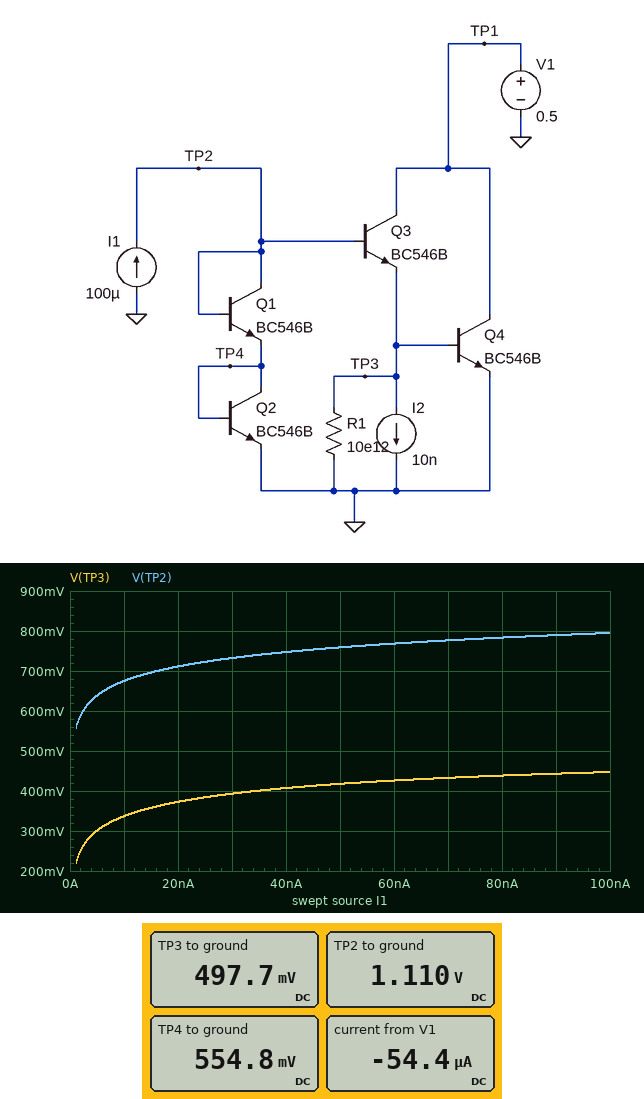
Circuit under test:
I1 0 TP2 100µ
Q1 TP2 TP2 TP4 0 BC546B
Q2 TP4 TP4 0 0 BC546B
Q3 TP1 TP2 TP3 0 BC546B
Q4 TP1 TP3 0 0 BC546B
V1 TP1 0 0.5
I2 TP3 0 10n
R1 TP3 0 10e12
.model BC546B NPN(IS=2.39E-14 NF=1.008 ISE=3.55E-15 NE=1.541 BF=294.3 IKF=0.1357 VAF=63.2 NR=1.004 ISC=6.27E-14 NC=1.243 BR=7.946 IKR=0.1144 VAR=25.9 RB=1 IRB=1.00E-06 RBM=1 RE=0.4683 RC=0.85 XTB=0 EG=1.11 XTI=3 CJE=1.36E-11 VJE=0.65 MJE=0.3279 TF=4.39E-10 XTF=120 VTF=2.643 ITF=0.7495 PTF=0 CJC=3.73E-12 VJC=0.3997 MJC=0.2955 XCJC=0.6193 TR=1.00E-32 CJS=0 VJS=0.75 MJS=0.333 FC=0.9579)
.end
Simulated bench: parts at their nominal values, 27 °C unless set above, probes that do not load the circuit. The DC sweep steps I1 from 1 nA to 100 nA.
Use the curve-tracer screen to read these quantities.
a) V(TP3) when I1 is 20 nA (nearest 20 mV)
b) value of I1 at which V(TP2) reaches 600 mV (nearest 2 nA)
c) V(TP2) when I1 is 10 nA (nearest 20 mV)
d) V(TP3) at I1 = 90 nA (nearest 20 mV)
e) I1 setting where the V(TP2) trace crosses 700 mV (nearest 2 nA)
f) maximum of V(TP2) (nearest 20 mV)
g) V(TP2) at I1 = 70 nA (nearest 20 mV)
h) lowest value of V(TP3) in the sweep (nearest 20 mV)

380 mV
2 nA
680 mV
440 mV
16 nA
800 mV
780 mV
220 mV
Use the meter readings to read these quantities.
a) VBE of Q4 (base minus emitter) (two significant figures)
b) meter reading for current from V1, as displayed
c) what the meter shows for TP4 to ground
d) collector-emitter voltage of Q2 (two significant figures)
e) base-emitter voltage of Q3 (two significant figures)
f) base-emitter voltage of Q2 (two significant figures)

500 mV
-54.4 µA
554.8 mV
550 mV
610 mV
550 mV
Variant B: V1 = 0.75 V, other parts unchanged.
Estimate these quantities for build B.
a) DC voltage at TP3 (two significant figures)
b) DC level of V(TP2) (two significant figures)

650 mV
1.2 V
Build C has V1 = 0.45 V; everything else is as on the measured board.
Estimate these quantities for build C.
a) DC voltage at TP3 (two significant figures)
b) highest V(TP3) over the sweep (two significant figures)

450 mV
430 mV
